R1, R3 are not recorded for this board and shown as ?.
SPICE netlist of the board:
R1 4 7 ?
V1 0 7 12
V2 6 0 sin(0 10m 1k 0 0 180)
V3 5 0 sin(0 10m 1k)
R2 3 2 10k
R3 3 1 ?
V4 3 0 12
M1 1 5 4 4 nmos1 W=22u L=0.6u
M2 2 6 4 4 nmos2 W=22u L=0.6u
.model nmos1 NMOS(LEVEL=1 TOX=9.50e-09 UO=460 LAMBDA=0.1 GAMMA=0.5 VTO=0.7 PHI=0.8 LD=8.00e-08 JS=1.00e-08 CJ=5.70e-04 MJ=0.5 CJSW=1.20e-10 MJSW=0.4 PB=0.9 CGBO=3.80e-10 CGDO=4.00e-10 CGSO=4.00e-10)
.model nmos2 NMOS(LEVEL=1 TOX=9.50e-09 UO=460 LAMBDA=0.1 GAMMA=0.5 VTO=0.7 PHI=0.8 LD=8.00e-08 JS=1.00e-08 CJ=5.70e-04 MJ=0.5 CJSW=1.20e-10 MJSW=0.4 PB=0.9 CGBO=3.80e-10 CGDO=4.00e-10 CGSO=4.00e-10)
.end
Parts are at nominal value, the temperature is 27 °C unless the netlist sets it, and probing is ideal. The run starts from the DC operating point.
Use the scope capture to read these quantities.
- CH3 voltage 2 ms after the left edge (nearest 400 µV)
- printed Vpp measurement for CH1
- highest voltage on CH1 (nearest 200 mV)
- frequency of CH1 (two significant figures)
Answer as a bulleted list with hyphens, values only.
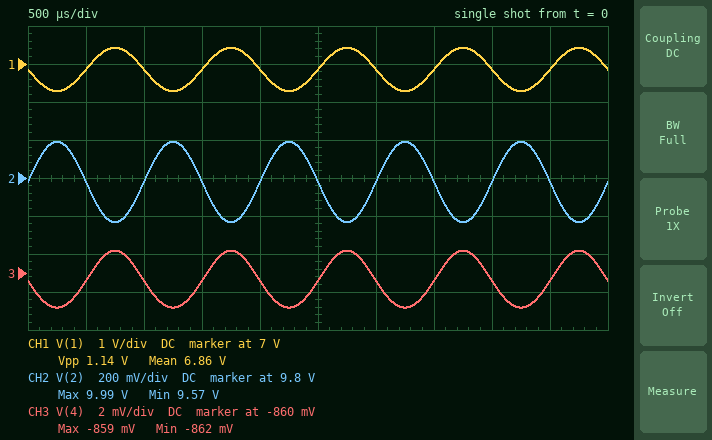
- -860.4 mV
- 1.14 V
- 7.4 V
- 1.0 kHz
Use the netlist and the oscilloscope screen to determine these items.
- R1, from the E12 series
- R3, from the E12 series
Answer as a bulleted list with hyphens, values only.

- 27 kΩ
- 27 kΩ
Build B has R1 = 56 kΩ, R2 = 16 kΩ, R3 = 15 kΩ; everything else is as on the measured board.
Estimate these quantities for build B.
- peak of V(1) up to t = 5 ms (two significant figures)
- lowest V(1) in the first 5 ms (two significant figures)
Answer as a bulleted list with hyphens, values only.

- 11 V
- 10 V
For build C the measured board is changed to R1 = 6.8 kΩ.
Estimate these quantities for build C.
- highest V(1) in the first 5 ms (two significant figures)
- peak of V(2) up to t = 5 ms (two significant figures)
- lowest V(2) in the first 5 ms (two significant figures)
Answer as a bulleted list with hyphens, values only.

- -1.0 V
- 920 mV
- 880 mV
